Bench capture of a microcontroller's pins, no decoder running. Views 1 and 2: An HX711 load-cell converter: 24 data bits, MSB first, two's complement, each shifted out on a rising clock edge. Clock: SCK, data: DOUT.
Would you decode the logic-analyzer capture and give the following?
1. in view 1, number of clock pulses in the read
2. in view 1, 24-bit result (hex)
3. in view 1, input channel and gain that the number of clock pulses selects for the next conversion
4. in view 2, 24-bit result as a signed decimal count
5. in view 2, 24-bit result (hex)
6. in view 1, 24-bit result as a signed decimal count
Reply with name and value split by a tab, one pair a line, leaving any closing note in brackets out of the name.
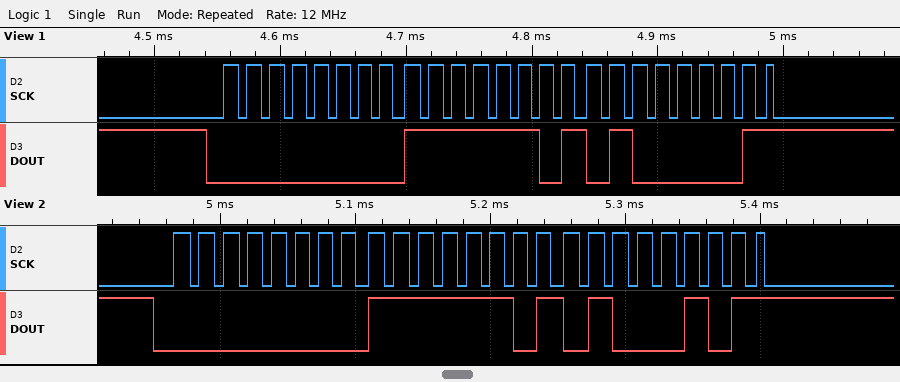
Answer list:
in view 1, number of clock pulses in the read	25
in view 1, 24-bit result	0x00FD41
in view 1, input channel and gain that the number of clock pulses selects for the next conversion	channel A, gain 128
in view 2, 24-bit result as a signed decimal count	64837
in view 2, 24-bit result	0x00FD45
in view 1, 24-bit result as a signed decimal count	64833
